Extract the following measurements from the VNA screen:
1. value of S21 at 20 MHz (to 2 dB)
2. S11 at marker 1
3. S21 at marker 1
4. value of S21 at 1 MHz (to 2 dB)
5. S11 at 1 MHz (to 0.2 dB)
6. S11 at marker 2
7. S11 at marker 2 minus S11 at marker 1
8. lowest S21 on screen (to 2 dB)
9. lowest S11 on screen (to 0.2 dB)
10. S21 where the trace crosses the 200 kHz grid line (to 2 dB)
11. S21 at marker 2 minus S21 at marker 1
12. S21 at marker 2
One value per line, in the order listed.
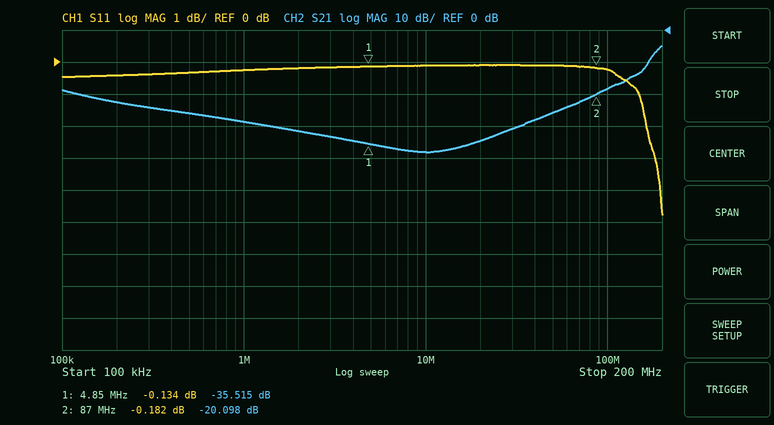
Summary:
-34 dB
-0.134 dB
-35.515 dB
-28 dB
-0.2 dB
-0.182 dB
-0.048 dB
-38 dB
-4.8 dB
-22 dB
15.417 dB
-20.098 dB
